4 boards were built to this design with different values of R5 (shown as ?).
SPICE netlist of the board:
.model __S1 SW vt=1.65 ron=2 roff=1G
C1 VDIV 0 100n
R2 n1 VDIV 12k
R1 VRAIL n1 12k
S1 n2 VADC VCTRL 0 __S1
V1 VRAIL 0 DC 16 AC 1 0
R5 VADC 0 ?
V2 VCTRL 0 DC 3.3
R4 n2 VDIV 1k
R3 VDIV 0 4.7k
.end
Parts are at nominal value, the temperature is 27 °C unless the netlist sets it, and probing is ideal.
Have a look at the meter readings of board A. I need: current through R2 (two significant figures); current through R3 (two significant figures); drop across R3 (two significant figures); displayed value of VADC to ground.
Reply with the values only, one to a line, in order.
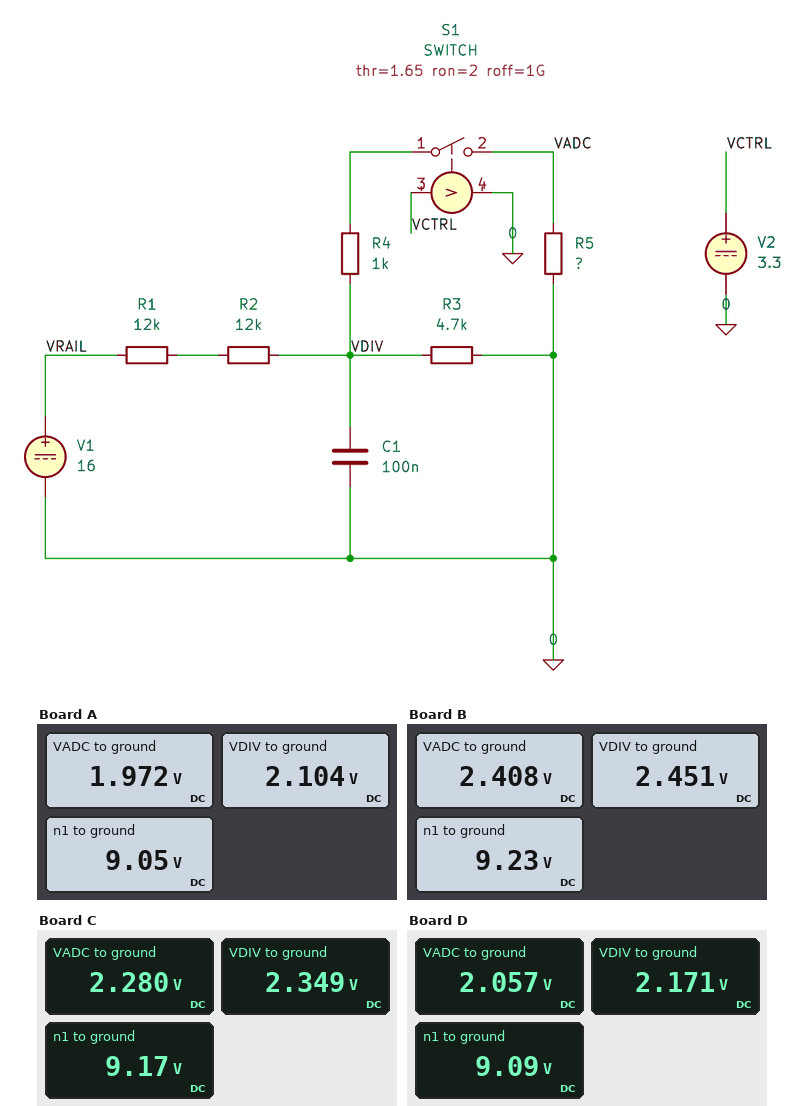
580 µA
450 µA
2.1 V
1.972 V
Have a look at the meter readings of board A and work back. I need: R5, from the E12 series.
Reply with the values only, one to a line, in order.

15 kΩ
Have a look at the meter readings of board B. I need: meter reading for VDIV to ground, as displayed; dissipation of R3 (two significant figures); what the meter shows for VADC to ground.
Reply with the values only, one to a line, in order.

2.451 V
1.3 mW
2.408 V
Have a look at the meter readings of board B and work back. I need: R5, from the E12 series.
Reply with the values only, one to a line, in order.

56 kΩ
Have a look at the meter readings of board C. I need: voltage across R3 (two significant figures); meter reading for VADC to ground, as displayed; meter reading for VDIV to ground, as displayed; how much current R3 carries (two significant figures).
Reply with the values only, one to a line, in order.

2.3 V
2.280 V
2.349 V
500 µA
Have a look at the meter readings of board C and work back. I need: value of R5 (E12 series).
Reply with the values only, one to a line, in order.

33 kΩ
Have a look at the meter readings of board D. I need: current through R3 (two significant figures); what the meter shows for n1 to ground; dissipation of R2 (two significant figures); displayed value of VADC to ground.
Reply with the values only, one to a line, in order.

460 µA
9.09 V
4.0 mW
2.057 V
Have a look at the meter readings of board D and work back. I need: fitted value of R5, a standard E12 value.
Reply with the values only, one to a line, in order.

18 kΩ
